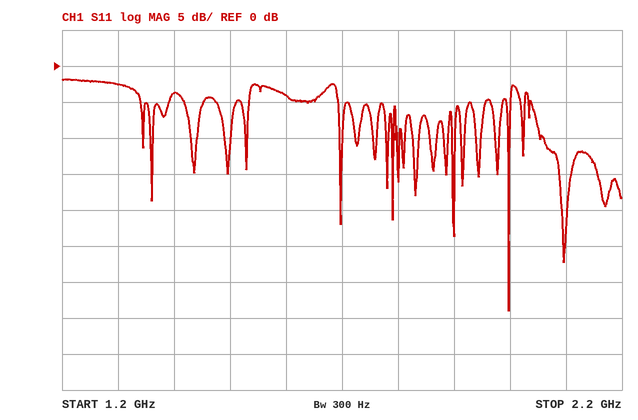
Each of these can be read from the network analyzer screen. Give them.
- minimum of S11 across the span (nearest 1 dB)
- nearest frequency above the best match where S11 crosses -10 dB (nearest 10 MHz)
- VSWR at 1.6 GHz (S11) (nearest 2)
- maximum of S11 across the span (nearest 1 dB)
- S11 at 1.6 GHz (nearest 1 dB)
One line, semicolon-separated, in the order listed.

-34 dB; 2.00 GHz; 4; -2 dB; -4 dB
